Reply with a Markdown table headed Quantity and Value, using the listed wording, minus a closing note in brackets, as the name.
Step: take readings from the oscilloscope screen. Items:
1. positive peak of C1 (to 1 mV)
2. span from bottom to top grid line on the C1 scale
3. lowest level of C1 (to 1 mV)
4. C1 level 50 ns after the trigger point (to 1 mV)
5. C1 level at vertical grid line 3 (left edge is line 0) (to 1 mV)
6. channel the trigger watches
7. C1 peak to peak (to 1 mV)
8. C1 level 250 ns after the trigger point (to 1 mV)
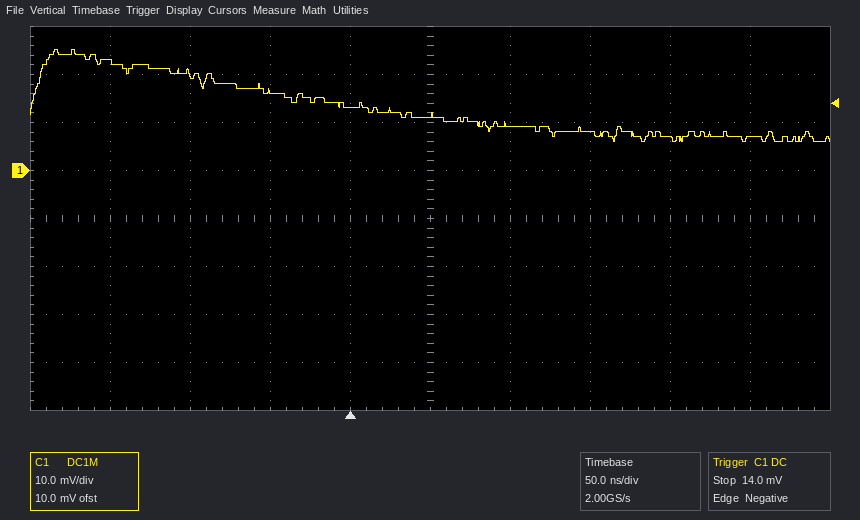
| Quantity | Value |
|---|---|
| positive peak of C1 | 25 mV |
| span from bottom to top grid line on the C1 scale | 80 mV |
| lowest level of C1 | 6 mV |
| C1 level 50 ns after the trigger point | 12 mV |
| C1 level at vertical grid line 3 (left edge is line 0) | 17 mV |
| channel the trigger watches | C1 |
| C1 peak to peak | 19 mV |
| C1 level 250 ns after the trigger point | 7 mV |
